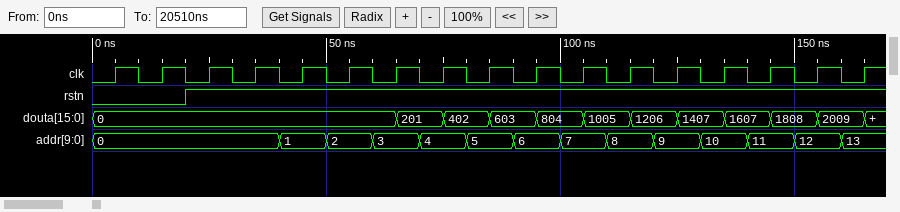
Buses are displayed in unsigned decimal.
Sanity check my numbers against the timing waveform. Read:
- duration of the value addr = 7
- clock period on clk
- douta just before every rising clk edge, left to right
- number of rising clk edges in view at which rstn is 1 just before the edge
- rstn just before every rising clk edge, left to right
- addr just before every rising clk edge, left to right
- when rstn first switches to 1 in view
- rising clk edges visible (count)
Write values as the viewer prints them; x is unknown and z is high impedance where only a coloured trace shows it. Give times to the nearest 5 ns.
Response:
10 ns
10 ns
0, 0, 0, 0, 0, 0, 0, 201, 402, 603, 804, 1005, 1206, 1407, 1607, 1808, 2009
15
0 0 1 1 1 1 1 1 1 1 1 1 1 1 1 1 1
0, 0, 0, 0, 1, 2, 3, 4, 5, 6, 7, 8, 9, 10, 11, 12, 13
20 ns
17
